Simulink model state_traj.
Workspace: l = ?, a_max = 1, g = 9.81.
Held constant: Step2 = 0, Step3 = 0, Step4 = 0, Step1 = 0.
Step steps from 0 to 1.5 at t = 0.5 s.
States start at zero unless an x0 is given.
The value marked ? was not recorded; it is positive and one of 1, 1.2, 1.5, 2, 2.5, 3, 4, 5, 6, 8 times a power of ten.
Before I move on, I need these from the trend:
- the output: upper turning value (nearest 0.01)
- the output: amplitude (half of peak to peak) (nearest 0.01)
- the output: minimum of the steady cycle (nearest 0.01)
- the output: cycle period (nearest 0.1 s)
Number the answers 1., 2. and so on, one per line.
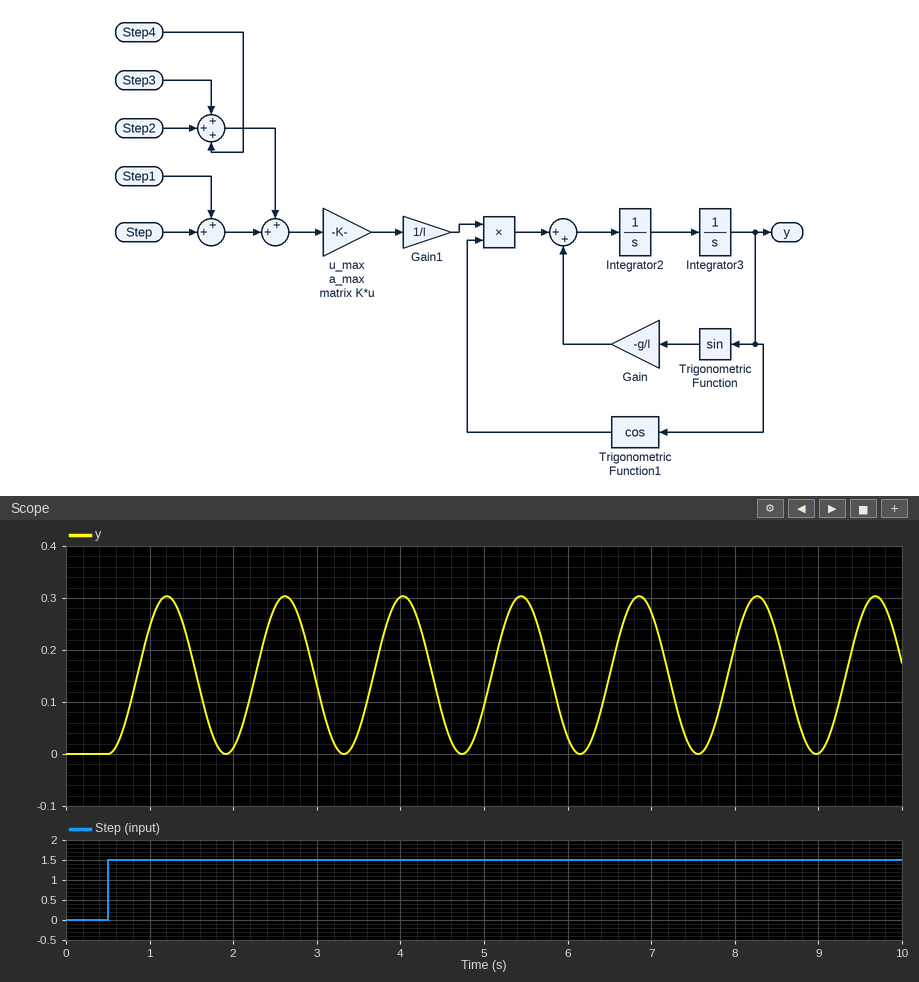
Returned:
1. 0.30
2. 0.15
3. 0.00
4. 1.4 s
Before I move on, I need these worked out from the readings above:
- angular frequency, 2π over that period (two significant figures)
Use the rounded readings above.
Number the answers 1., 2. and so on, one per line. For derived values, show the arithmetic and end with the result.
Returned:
1. 2π / 1.4 = 4.5 rad/s
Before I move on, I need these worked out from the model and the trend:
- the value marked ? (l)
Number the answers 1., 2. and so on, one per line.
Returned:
1. 0.5
